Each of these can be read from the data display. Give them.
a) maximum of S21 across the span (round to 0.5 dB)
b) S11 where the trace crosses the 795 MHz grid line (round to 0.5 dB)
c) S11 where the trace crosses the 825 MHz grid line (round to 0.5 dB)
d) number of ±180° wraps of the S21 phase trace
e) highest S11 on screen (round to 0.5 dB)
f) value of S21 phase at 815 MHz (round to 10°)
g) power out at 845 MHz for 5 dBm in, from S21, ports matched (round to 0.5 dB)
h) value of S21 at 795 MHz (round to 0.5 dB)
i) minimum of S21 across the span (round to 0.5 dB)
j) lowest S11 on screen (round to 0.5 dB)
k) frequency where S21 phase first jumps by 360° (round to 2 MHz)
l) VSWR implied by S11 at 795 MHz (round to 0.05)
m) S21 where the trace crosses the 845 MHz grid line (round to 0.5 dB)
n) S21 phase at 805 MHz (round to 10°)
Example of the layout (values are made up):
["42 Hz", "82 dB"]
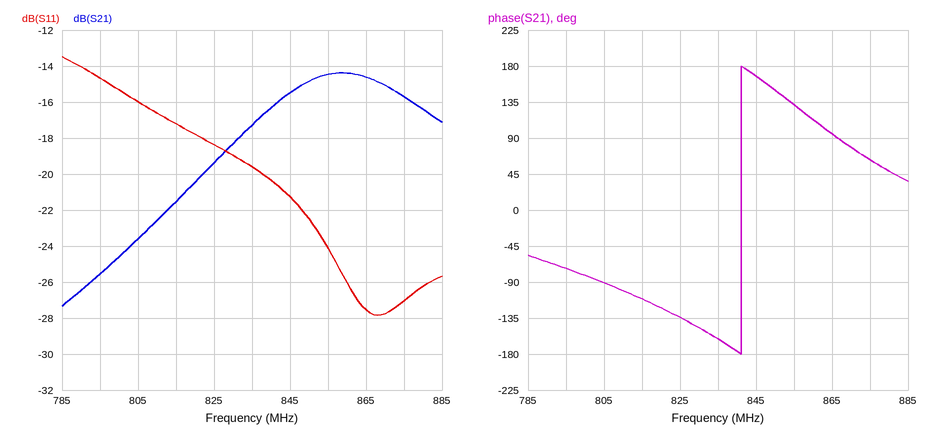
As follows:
["-14.5 dB", "-14.5 dB", "-18.5 dB", "1", "-13.5 dB", "-110°", "-10.5 dBm", "-25.5 dB", "-27.5 dB", "-28.0 dB", "842 MHz", "1.45", "-15.5 dB", "-90°"]
